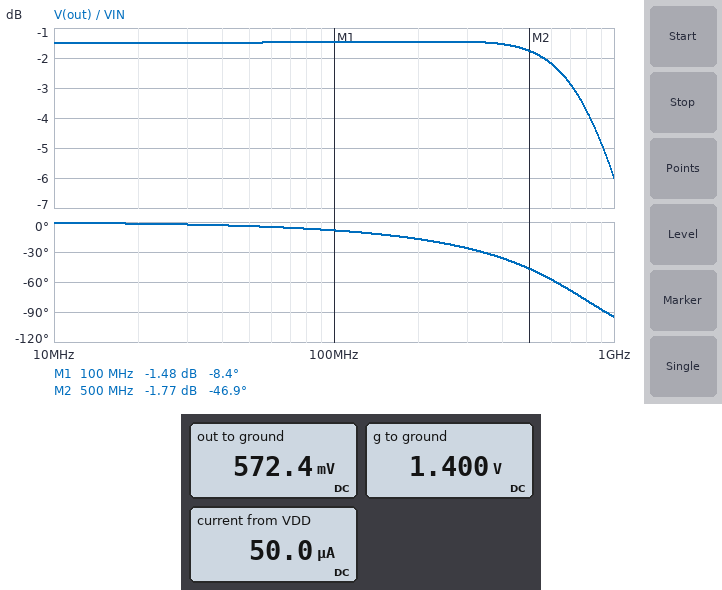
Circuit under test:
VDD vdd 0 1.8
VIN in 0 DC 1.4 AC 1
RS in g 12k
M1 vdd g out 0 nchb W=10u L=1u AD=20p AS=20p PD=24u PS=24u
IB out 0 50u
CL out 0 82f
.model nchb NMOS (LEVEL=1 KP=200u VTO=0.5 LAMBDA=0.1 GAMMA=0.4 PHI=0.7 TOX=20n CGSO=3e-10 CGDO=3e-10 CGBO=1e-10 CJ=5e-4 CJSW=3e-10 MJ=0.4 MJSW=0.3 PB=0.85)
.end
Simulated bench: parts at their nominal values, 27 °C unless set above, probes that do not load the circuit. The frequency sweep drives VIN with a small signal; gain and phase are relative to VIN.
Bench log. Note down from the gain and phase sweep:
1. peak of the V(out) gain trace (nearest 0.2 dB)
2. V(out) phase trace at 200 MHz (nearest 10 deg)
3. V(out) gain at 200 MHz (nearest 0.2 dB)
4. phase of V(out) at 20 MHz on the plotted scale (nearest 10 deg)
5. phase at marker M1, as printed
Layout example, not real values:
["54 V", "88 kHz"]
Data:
["-1.4 dB", "-20 deg", "-1.4 dB", "0 deg", "-8.4 deg"]
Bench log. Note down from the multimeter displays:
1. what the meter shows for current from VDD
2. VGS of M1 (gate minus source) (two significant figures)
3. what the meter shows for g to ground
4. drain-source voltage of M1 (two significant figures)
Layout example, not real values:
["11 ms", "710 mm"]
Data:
["50.0 µA", "830 mV", "1.400 V", "1.2 V"]
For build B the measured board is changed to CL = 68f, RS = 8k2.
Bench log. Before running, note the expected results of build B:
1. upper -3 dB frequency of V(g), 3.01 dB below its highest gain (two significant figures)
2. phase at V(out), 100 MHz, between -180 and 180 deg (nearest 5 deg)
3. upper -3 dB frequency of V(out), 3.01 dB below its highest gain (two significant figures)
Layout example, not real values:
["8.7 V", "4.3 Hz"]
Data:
["1.6 GHz", "-5 deg", "1.1 GHz"]
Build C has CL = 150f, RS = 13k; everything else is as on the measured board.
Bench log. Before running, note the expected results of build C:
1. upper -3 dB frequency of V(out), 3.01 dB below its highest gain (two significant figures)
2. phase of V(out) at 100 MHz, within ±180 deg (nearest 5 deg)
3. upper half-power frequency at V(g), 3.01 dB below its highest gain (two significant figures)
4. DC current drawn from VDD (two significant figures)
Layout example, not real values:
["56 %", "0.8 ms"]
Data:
["580 MHz", "-15 deg", "930 MHz", "50 µA"]
